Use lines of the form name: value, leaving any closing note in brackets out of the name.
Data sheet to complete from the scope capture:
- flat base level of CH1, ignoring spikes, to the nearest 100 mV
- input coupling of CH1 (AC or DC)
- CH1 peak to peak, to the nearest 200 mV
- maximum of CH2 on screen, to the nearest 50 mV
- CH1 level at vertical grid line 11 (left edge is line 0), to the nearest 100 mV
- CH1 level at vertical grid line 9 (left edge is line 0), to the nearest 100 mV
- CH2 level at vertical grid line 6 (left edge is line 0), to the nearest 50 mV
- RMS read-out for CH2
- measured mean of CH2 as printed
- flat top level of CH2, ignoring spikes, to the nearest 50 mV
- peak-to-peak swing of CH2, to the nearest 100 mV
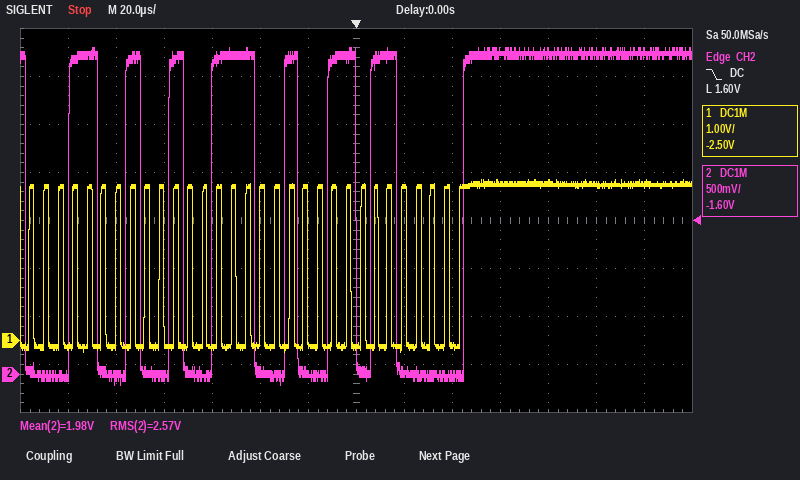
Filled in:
flat base level of CH1, ignoring spikes, to the nearest 100 mV: -100 mV
input coupling of CH1: DC
CH1 peak to peak, to the nearest 200 mV: 3.6 V
maximum of CH2 on screen, to the nearest 50 mV: 3.40 V
CH1 level at vertical grid line 11 (left edge is line 0), to the nearest 100 mV: 3.3 V
CH1 level at vertical grid line 9 (left edge is line 0), to the nearest 100 mV: -100 mV
CH2 level at vertical grid line 6 (left edge is line 0), to the nearest 50 mV: 0 mV
RMS read-out for CH2: 2.57 V
measured mean of CH2 as printed: 1.98 V
flat top level of CH2, ignoring spikes, to the nearest 50 mV: 3.30 V
peak-to-peak swing of CH2, to the nearest 100 mV: 3.50 V
